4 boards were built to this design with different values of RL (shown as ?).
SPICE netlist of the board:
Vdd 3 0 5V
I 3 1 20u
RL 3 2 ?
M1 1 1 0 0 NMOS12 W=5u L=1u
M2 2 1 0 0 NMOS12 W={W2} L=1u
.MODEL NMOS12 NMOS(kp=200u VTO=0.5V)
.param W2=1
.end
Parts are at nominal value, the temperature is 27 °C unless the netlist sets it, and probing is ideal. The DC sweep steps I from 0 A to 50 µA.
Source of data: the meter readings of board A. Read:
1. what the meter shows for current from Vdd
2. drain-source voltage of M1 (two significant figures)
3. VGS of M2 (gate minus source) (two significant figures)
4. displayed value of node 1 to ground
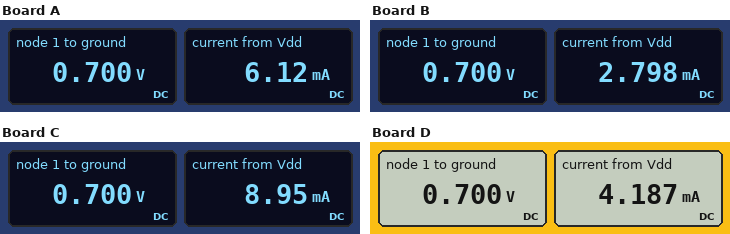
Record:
6.12 mA
700 mV
700 mV
0.700 V
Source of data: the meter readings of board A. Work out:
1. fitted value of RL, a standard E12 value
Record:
820 Ω
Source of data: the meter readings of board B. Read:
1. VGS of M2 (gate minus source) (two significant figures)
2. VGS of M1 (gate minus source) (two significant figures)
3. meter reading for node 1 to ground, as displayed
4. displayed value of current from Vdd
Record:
700 mV
700 mV
0.700 V
2.798 mA
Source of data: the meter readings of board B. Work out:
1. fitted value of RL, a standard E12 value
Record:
1.8 kΩ
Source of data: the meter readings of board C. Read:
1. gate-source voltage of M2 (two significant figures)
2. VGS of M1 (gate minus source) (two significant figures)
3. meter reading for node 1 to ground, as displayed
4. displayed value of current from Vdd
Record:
700 mV
700 mV
0.700 V
8.95 mA
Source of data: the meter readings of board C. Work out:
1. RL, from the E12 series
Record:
560 Ω
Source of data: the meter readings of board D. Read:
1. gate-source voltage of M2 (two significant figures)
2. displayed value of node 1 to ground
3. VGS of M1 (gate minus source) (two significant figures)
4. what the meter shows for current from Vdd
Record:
700 mV
0.700 V
700 mV
4.187 mA
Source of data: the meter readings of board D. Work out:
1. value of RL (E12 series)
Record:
1.2 kΩ
